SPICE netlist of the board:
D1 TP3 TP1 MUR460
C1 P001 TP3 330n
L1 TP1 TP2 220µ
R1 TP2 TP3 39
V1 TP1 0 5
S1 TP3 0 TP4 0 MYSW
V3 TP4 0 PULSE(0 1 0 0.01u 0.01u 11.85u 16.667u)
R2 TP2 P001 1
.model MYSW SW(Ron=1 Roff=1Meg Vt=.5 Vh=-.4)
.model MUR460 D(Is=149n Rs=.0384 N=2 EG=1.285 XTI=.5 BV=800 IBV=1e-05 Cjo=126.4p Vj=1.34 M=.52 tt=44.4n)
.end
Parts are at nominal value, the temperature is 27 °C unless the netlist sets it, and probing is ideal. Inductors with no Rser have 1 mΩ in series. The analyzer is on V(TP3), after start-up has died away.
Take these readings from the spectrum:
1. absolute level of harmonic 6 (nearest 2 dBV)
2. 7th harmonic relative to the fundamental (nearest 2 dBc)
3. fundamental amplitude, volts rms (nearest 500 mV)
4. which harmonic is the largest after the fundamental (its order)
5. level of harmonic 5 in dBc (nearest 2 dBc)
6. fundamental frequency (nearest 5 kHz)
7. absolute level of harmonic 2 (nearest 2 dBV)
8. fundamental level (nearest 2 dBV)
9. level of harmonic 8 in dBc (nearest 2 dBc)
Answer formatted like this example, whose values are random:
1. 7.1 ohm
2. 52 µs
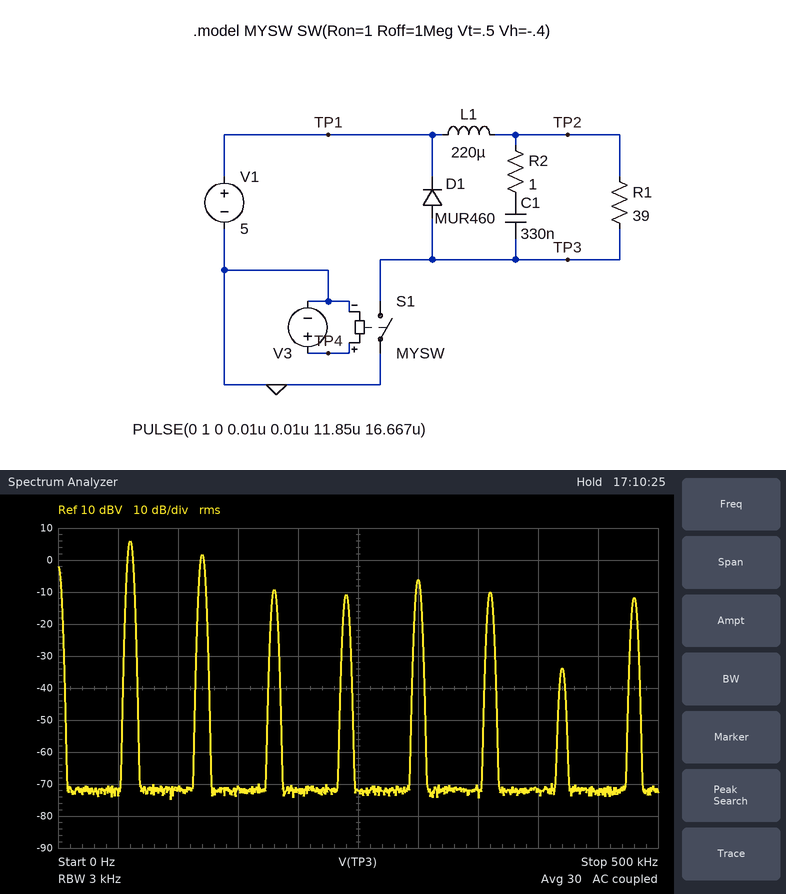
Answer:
1. -10 dBV
2. -40 dBc
3. 2.0 V
4. 2
5. -12 dBc
6. 60 kHz
7. 2 dBV
8. 6 dBV
9. -18 dBc
